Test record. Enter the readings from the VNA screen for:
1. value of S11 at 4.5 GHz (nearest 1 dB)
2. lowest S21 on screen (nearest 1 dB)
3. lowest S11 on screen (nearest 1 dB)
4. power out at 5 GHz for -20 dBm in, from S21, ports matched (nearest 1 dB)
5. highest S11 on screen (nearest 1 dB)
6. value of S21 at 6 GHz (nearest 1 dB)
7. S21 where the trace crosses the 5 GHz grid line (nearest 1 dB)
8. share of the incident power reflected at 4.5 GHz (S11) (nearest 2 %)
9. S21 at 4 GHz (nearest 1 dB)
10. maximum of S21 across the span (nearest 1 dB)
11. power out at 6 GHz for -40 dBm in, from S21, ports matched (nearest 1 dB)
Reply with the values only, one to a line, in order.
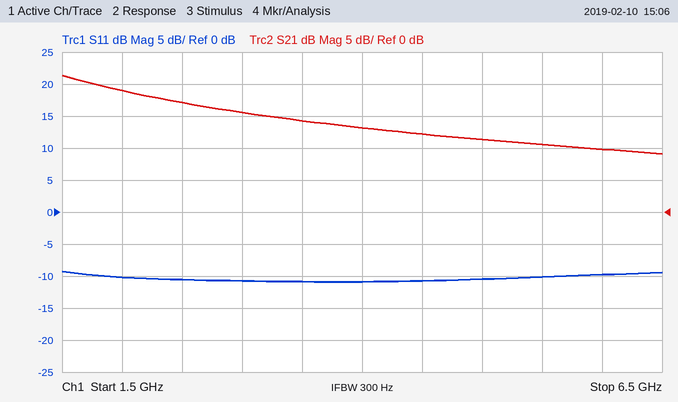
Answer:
-11 dB
9 dB
-11 dB
-9 dBm
-9 dB
10 dB
11 dB
8 %
13 dB
21 dB
-30 dBm
